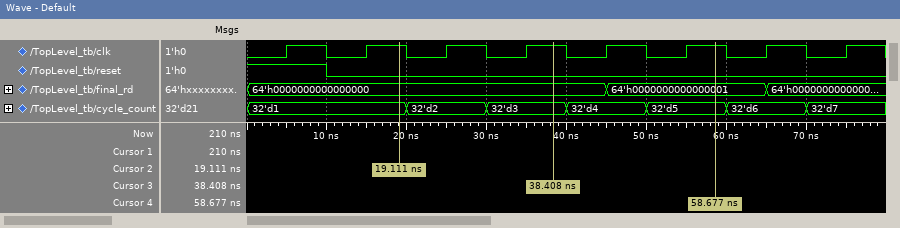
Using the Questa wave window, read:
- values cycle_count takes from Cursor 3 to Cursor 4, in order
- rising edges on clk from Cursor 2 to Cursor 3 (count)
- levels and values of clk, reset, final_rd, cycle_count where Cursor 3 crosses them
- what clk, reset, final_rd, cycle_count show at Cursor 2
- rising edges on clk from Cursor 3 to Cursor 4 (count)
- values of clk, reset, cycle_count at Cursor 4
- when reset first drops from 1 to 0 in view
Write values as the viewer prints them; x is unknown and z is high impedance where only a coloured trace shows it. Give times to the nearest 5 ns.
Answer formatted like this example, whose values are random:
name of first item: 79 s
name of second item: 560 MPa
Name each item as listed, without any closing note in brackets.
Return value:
values cycle_count takes from Cursor 3 to Cursor 4, in order: 32'd3, 32'd4, 32'd5
rising edges on clk from Cursor 2 to Cursor 3: 2
levels and values of clk, reset, final_rd, cycle_count where Cursor 3 crosses them: clk=1, reset=0, final_rd=64'h0000000000000000, cycle_count=32'd3
what clk, reset, final_rd, cycle_count show at Cursor 2: clk=1, reset=0, final_rd=64'h0000000000000000, cycle_count=32'd1
rising edges on clk from Cursor 3 to Cursor 4: 2
values of clk, reset, cycle_count at Cursor 4: clk=1, reset=0, cycle_count=32'd5
when reset first drops from 1 to 0 in view: 10 ns
